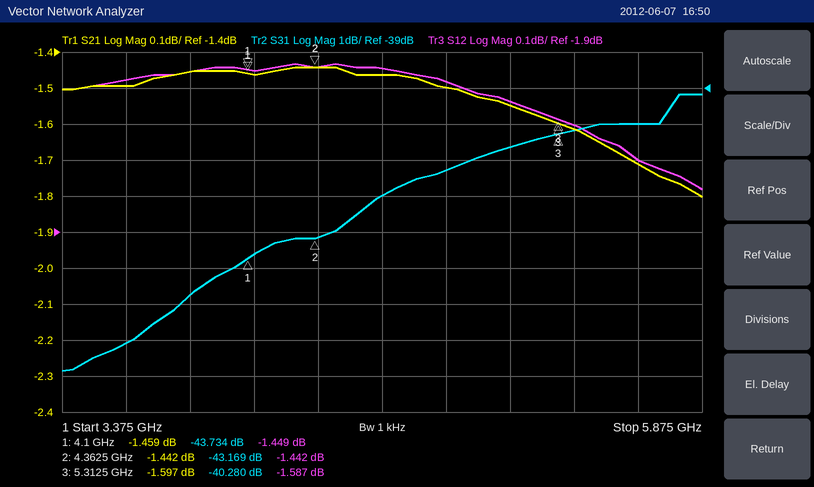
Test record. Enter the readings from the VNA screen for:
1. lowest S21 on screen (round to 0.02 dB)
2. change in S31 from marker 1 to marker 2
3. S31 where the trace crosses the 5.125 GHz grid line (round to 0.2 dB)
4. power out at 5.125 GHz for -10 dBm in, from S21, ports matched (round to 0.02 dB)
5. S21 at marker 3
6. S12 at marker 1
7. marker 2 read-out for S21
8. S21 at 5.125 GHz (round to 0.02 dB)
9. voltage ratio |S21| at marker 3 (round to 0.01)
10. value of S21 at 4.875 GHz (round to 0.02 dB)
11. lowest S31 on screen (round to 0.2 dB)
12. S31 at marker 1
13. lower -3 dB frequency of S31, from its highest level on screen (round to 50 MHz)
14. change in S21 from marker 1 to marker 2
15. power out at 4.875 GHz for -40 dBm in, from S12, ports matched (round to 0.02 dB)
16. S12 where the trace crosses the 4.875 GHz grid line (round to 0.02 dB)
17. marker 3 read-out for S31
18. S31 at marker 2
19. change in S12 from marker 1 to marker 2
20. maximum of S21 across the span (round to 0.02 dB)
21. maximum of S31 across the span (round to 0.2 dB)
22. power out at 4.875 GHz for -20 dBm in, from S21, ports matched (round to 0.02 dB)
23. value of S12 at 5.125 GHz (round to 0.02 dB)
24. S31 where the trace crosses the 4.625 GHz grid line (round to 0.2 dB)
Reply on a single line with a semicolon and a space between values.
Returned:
-1.80 dB; 0.565 dB; -40.6 dB; -11.54 dBm; -1.597 dB; -1.449 dB; -1.442 dB; -1.54 dB; 0.83; -1.50 dB; -46.8 dB; -43.734 dB; 4.60 GHz; 0.017 dB; -41.48 dBm; -1.48 dB; -40.280 dB; -43.169 dB; 0.007 dB; -1.44 dB; -39.2 dB; -21.50 dBm; -1.54 dB; -42.0 dB
